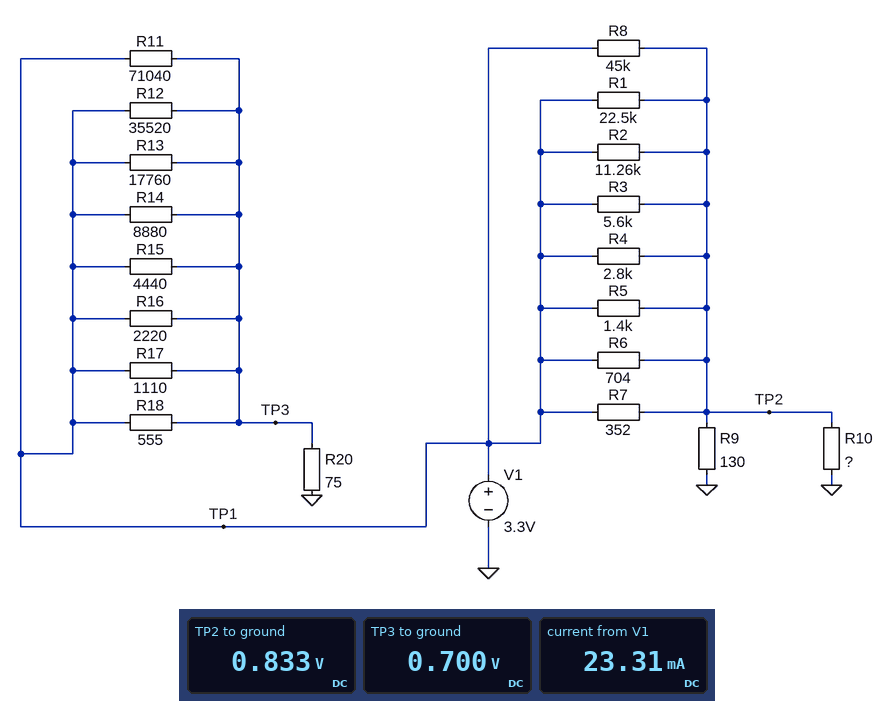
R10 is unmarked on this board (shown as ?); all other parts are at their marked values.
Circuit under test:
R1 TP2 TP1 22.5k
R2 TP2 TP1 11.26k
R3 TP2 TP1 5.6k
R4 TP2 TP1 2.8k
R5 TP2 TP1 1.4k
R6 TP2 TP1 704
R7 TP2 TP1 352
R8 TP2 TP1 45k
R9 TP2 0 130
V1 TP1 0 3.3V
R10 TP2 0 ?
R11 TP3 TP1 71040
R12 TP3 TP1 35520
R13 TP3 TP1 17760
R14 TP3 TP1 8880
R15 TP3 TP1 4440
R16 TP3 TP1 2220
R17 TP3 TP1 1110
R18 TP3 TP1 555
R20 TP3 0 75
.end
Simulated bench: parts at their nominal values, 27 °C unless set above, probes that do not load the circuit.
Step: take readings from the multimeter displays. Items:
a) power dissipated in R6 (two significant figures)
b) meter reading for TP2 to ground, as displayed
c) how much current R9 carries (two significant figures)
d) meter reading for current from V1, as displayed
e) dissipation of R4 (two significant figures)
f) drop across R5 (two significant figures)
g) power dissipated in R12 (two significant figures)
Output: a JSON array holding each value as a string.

["8.6 mW", "0.833 V", "6.4 mA", "23.31 mA", "2.2 mW", "2.5 V", "190 µW"]
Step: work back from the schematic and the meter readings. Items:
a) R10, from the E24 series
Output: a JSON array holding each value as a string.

["110 Ω"]
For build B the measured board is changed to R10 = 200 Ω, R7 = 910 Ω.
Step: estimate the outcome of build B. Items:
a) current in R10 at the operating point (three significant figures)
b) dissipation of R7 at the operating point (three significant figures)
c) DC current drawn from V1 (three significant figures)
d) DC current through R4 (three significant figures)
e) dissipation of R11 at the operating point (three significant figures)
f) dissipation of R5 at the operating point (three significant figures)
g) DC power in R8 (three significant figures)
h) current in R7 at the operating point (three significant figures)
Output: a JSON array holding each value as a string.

["3.90 mA", "6.98 mW", "19.2 mA", "900 µA", "95.2 µW", "4.54 mW", "141 µW", "2.77 mA"]
